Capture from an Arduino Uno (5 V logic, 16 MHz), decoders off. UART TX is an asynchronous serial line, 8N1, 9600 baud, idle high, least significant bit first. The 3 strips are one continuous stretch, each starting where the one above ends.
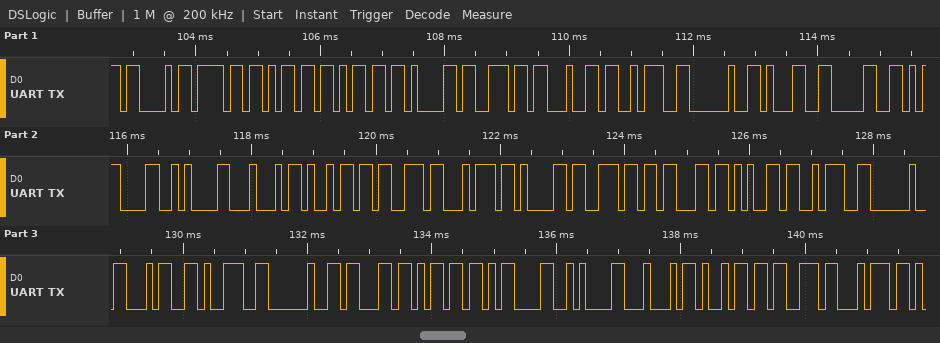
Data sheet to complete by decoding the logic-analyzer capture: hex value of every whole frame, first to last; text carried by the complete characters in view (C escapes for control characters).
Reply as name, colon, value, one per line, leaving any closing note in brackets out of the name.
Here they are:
hex value of every whole frame, first to last: 43 6F 6D 6D 61 6E 64 3A 20 31 30 0D 0A 44 69 73 74 61 6E 63 65 3A 20 34 39 20 63 6D 0D 0A 44 69 73 74
text carried by the complete characters in view: "Command: 10\r\nDistance: 49 cm\r\nDist"
